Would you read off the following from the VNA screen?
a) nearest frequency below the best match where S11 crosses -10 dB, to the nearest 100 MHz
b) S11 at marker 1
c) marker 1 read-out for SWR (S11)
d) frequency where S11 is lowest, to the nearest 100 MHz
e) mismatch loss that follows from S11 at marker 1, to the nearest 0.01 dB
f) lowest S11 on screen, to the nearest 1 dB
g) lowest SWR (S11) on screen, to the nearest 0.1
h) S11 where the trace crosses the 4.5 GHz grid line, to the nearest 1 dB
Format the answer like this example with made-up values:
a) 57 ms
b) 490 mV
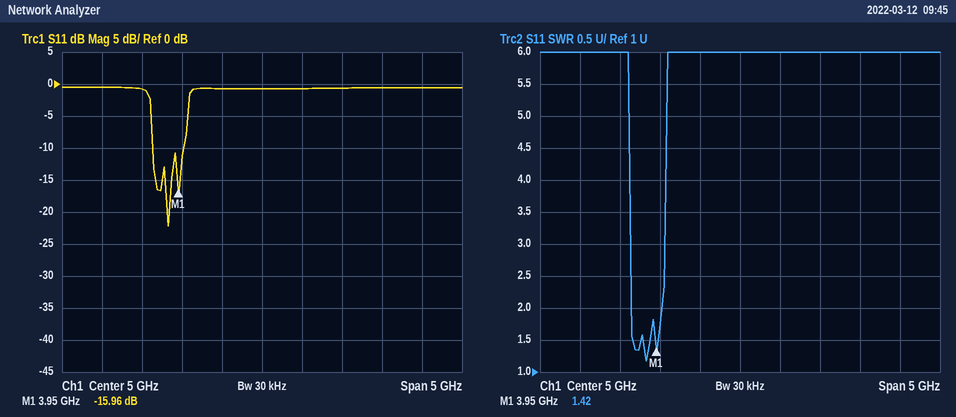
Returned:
a) 3.6 GHz
b) -15.96 dB
c) 1.42
d) 3.8 GHz
e) 0.11 dB
f) -22 dB
g) 1.2
h) -1 dB
